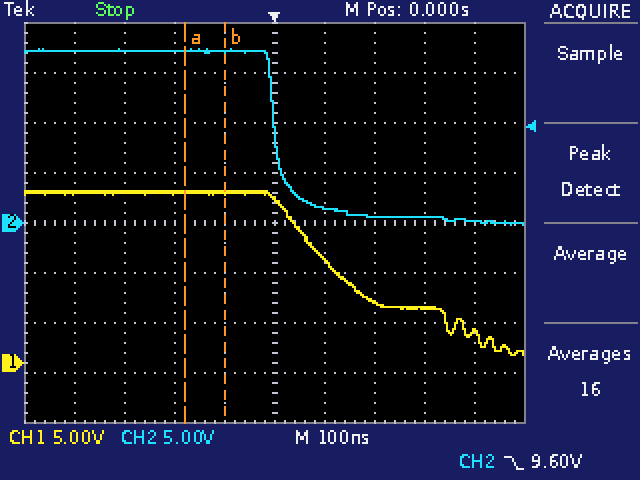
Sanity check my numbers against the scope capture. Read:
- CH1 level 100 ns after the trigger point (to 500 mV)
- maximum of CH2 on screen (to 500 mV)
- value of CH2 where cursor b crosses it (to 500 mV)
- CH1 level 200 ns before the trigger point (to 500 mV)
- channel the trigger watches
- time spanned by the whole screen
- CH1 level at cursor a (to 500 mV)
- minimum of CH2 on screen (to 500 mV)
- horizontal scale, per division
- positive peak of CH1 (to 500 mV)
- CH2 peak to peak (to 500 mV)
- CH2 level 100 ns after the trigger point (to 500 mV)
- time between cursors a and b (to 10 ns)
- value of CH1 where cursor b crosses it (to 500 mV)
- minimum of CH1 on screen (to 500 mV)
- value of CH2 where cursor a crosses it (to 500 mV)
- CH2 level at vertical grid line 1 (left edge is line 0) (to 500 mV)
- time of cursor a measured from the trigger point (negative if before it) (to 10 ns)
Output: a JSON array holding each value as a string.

["10.5 V", "17.5 V", "17.0 V", "17.0 V", "CH2", "1 µs", "17.0 V", "0.0 V", "100 ns", "17.0 V", "17.5 V", "1.5 V", "80 ns", "17.0 V", "1.0 V", "17.0 V", "17.0 V", "-180 ns"]
